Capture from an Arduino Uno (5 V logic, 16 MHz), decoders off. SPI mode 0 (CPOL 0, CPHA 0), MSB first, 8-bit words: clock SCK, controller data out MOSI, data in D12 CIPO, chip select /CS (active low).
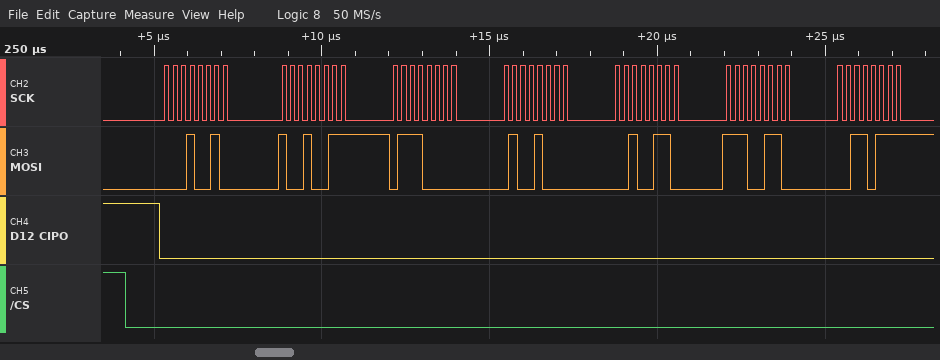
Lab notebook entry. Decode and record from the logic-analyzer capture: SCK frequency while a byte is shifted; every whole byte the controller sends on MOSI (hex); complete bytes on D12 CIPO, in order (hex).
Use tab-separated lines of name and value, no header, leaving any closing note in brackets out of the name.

SCK frequency while a byte is shifted	4 MHz
every whole byte the controller sends on MOSI	12 93 70 48 26 E6 37
complete bytes on D12 CIPO, in order	00 00 00 00 00 00 00
